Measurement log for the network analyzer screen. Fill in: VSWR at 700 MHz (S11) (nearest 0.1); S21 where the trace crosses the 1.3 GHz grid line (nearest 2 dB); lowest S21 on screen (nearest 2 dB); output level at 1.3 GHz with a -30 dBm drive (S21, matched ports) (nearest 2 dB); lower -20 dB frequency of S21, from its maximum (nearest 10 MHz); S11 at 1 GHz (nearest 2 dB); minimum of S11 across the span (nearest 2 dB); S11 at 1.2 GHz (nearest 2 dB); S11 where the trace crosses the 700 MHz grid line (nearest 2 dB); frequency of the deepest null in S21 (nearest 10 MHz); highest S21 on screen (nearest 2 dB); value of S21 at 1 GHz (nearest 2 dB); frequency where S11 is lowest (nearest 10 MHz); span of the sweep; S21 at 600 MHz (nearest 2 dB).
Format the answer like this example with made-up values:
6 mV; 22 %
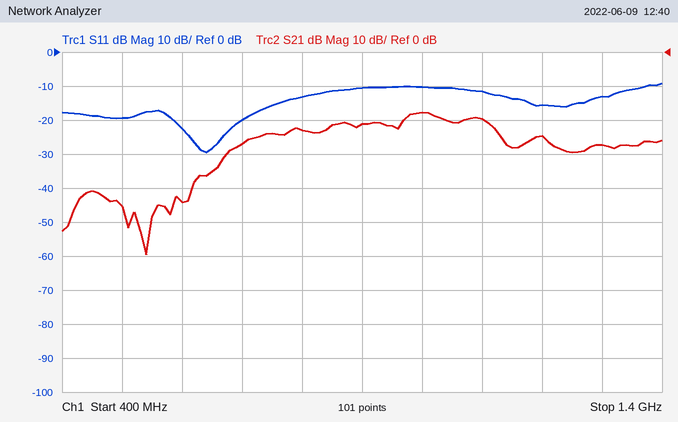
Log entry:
1.2; -28 dB; -60 dB; -58 dBm; 620 MHz; -10 dB; -30 dB; -16 dB; -20 dB; 540 MHz; -18 dB; -18 dB; 640 MHz; 1 GHz; -44 dB
